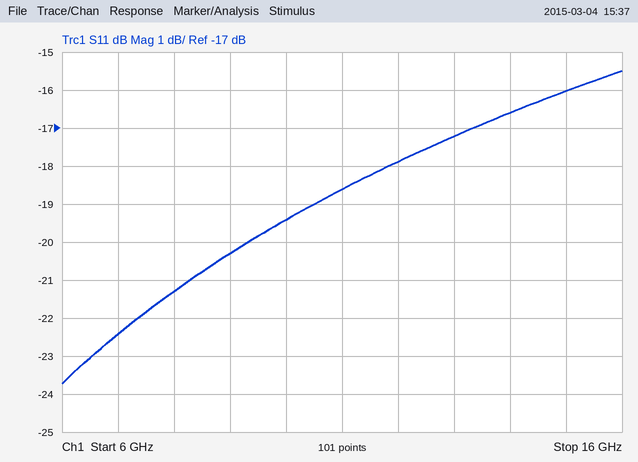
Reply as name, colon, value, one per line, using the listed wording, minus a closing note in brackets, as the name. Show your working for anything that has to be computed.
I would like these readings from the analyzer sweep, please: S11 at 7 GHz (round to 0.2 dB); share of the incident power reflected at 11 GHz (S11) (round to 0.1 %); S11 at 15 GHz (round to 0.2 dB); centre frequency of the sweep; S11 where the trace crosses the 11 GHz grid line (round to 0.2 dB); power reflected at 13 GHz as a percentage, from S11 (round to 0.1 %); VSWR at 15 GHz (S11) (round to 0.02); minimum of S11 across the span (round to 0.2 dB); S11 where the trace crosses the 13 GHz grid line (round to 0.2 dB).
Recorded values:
S11 at 7 GHz: -22.4 dB
share of the incident power reflected at 11 GHz (S11): 10^(-18.6/10) ≈ 1.4 %
S11 at 15 GHz: -16.0 dB
centre frequency of the sweep: 11 GHz
S11 where the trace crosses the 11 GHz grid line: -18.6 dB
power reflected at 13 GHz as a percentage, from S11: 10^(-17.2/10) ≈ 1.9 %
VSWR at 15 GHz (S11): |Γ| = 10^(-16/20) = 0.1585; VSWR = (1 + 0.1585)/(1 − 0.1585) ≈ 1.38
minimum of S11 across the span: -23.8 dB
S11 where the trace crosses the 13 GHz grid line: -17.2 dB
